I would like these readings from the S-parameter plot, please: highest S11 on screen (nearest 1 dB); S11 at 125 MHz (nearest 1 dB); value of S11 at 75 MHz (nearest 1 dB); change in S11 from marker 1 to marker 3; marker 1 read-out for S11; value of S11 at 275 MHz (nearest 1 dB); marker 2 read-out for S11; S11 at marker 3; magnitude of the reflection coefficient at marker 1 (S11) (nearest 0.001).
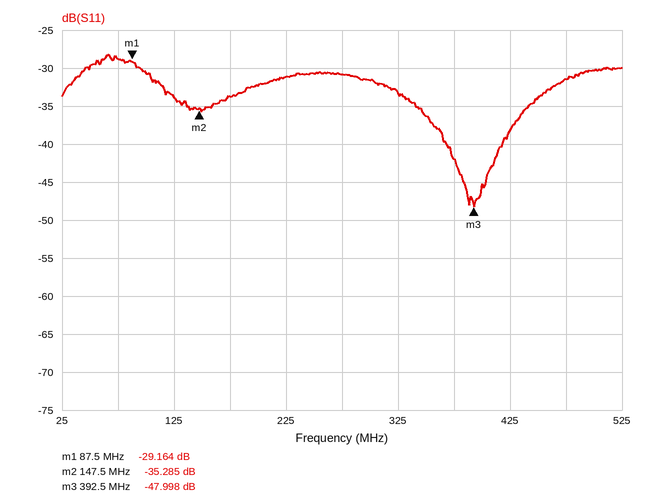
-28 dB
-34 dB
-29 dB
-18.834 dB
-29.164 dB
-31 dB
-35.285 dB
-47.998 dB
0.035
